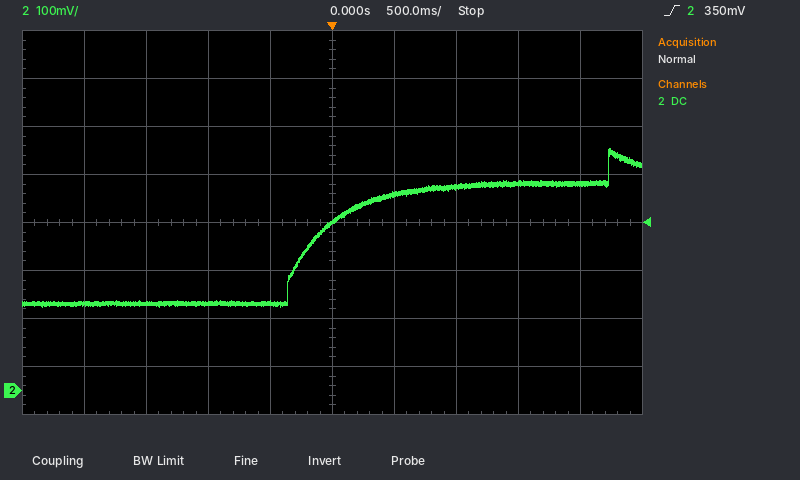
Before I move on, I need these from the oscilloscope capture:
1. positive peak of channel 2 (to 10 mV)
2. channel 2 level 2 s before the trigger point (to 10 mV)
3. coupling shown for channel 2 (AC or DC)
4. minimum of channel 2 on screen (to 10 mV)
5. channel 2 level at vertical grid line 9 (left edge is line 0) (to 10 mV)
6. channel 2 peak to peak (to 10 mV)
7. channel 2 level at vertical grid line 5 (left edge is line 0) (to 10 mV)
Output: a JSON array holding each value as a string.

["500 mV", "180 mV", "DC", "170 mV", "430 mV", "330 mV", "350 mV"]
